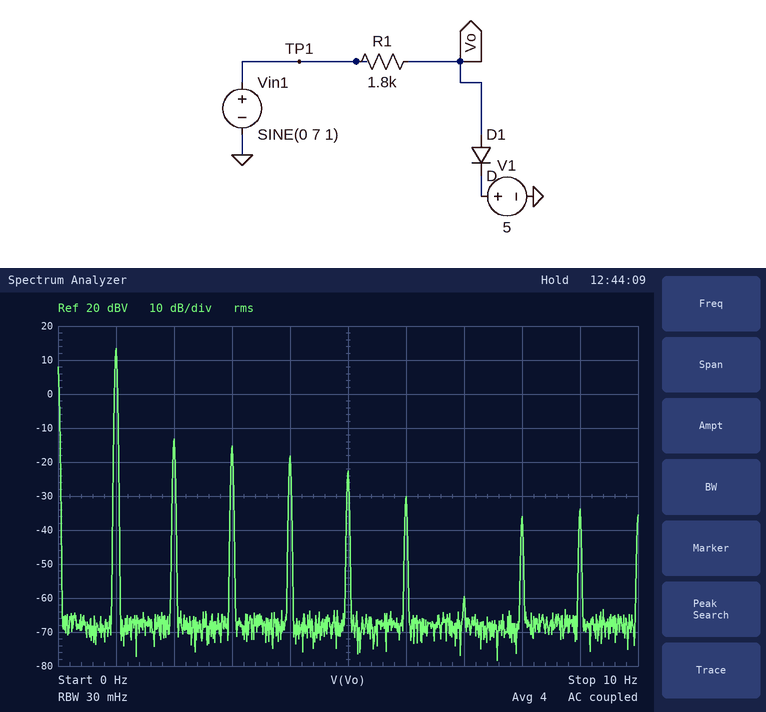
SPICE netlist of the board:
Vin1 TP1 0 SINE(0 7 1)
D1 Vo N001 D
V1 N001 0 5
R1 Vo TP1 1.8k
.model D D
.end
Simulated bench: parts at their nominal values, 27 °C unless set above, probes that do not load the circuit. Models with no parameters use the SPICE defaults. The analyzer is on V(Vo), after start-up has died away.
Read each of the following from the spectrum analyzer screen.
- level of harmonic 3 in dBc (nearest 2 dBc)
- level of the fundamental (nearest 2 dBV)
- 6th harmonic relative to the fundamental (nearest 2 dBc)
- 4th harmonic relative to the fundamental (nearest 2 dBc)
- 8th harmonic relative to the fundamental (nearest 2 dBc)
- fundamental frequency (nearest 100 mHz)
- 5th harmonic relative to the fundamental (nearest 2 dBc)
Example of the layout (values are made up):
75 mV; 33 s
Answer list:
-28 dBc; 14 dBV; -44 dBc; -32 dBc; -50 dBc; 1.0 Hz; -36 dBc
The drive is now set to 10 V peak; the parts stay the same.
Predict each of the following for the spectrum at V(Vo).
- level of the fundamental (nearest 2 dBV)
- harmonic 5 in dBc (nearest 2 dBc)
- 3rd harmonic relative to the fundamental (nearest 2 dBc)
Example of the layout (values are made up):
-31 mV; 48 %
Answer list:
16 dBV; -42 dBc; -22 dBc
